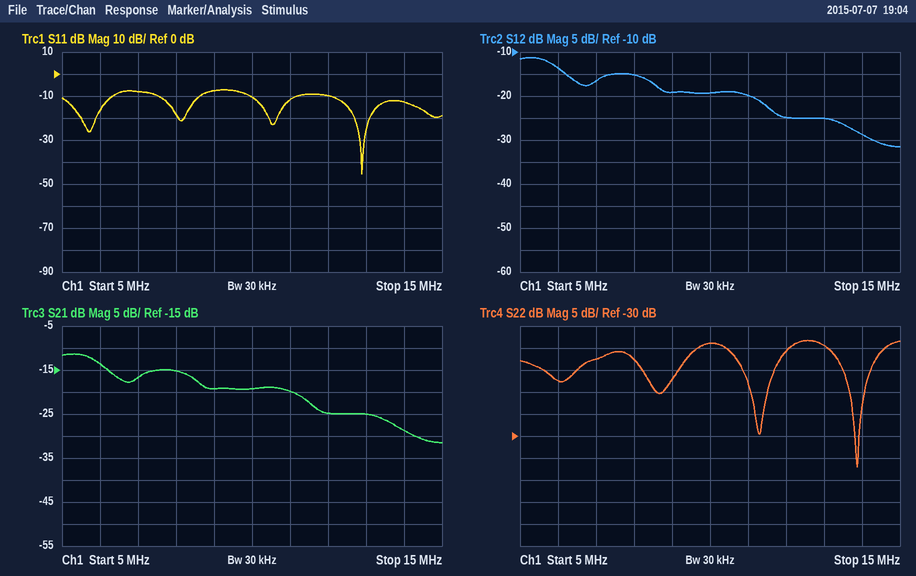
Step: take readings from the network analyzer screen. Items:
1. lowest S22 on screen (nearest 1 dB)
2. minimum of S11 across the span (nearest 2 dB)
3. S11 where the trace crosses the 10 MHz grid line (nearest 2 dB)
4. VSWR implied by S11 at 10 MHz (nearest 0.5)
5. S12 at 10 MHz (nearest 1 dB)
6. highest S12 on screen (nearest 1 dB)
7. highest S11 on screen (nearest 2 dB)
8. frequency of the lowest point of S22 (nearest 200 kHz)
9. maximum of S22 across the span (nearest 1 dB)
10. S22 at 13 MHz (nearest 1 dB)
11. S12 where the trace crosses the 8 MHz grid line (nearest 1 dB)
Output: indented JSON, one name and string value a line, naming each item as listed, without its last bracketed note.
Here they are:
{
  "lowest S22 on screen": "-37 dB",
  "minimum of S11 across the span": "-46 dB",
  "S11 where the trace crosses the 10 MHz grid line": "-10 dB",
  "VSWR implied by S11 at 10 MHz": "2.0",
  "S12 at 10 MHz": "-19 dB",
  "highest S12 on screen": "-11 dB",
  "highest S11 on screen": "-8 dB",
  "frequency of the lowest point of S22": "13.8 MHz",
  "maximum of S22 across the span": "-8 dB",
  "S22 at 13 MHz": "-9 dB",
  "S12 where the trace crosses the 8 MHz grid line": "-15 dB"
}
